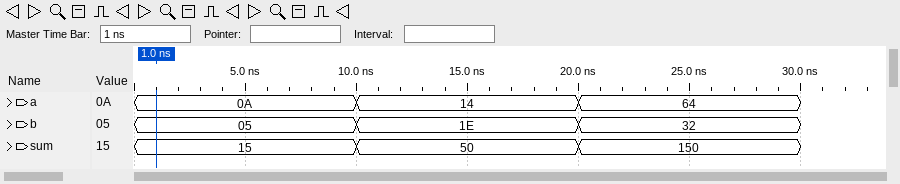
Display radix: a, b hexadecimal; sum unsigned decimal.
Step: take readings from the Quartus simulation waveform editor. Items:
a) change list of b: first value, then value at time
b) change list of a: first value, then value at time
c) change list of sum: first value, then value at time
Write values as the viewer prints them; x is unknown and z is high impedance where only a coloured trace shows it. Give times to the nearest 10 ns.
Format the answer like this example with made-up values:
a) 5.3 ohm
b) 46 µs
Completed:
a) 05, 1E at 10 ns, 32 at 20 ns
b) 0A, 14 at 10 ns, 64 at 20 ns
c) 15, 50 at 10 ns, 150 at 20 ns
